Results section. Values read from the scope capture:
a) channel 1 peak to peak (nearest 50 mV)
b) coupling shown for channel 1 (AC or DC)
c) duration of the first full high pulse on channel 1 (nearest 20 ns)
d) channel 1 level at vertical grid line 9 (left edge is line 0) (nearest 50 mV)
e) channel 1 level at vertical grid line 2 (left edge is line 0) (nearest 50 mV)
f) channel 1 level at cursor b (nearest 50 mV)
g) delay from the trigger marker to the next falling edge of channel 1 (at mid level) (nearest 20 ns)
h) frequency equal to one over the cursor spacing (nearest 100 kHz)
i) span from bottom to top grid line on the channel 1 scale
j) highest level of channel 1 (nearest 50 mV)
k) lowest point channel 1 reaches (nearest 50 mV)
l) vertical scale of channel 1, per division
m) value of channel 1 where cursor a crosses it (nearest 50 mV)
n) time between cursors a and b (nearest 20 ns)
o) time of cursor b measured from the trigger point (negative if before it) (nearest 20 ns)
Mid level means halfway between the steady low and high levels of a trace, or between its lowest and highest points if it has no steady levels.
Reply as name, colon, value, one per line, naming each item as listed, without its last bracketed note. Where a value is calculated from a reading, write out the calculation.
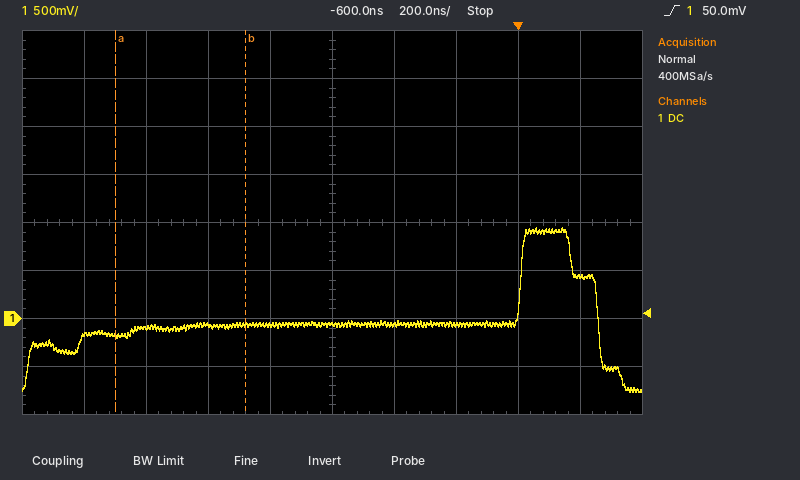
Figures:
channel 1 peak to peak: 950 mV − (-750 mV) = 1.70 V
coupling shown for channel 1: DC
duration of the first full high pulse on channel 1: 260 ns
channel 1 level at vertical grid line 9 (left edge is line 0): 450 mV
channel 1 level at vertical grid line 2 (left edge is line 0): -100 mV
channel 1 level at cursor b: -50 mV
delay from the trigger marker to the next falling edge of channel 1 (at mid level): 260 ns
frequency equal to one over the cursor spacing: 1 / 420 ns ≈ 2.4 MHz
span from bottom to top grid line on the channel 1 scale: 4 V
highest level of channel 1: 950 mV
lowest point channel 1 reaches: -750 mV
vertical scale of channel 1, per division: 500 mV
value of channel 1 where cursor a crosses it: -200 mV
time between cursors a and b: 420 ns
time of cursor b measured from the trigger point (negative if before it): -880 ns
